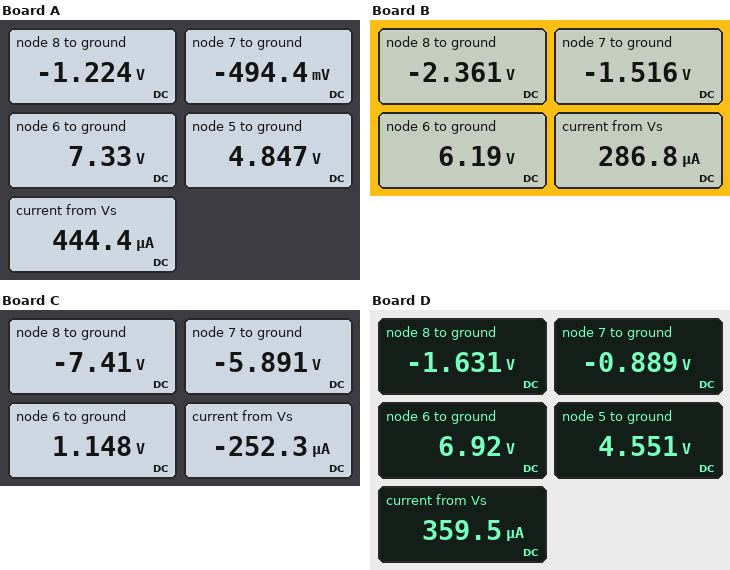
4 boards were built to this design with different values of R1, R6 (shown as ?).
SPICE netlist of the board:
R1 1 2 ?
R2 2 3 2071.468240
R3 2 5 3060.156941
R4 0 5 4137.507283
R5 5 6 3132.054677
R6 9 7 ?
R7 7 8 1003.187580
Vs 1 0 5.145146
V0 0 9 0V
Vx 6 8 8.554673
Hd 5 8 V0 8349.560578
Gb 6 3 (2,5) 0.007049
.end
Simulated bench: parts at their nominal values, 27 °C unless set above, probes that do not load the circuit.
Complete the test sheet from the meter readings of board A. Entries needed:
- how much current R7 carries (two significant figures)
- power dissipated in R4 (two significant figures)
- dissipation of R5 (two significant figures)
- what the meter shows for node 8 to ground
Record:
730 µA
5.7 mW
2.0 mW
-1.224 V
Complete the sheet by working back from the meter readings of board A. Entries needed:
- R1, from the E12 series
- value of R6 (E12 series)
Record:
820 Ω
680 Ω
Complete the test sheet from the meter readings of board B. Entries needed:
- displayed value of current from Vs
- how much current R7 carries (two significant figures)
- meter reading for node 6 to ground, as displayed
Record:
286.8 µA
840 µA
6.19 V
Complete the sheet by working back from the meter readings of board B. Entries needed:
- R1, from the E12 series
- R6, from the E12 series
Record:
1.8 kΩ
1.8 kΩ
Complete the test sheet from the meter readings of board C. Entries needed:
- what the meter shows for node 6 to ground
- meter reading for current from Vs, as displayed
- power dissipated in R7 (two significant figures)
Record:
1.148 V
-252.3 µA
2.3 mW
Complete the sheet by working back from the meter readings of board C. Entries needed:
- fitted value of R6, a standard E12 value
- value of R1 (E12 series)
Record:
3.9 kΩ
390 Ω
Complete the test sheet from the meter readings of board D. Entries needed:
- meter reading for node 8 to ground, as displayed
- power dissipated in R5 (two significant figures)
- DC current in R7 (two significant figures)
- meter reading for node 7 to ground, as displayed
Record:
-1.631 V
1.8 mW
740 µA
-0.889 V
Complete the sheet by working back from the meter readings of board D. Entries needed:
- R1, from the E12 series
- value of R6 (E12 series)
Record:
1.8 kΩ
1.2 kΩ
